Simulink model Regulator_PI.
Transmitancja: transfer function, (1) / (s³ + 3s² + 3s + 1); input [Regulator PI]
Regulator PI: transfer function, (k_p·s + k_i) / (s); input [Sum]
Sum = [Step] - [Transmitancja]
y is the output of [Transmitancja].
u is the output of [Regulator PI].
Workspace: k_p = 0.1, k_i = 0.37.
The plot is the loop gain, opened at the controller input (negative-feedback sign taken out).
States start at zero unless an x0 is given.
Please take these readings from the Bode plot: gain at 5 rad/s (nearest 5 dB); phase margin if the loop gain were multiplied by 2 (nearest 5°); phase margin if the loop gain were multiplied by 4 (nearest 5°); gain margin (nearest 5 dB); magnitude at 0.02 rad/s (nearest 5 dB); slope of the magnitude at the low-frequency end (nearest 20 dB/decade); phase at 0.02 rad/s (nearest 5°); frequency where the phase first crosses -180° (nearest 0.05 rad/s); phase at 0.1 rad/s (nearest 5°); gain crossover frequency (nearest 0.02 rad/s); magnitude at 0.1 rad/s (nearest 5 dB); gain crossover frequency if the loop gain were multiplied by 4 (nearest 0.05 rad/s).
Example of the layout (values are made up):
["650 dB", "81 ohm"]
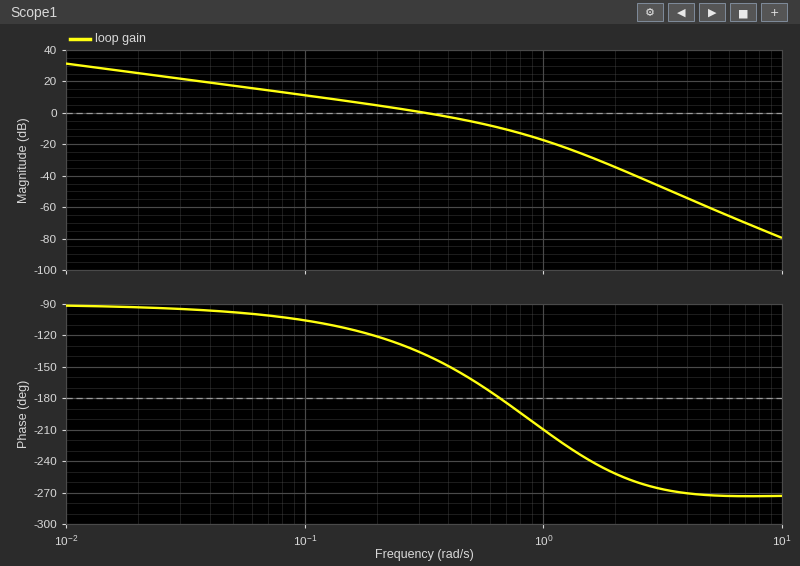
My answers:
["-60 dB", "15°", "-10°", "10 dB", "25 dB", "-20 dB/decade", "-95°", "0.65 rad/s", "-105°", "0.32 rad/s", "10 dB", "0.75 rad/s"]
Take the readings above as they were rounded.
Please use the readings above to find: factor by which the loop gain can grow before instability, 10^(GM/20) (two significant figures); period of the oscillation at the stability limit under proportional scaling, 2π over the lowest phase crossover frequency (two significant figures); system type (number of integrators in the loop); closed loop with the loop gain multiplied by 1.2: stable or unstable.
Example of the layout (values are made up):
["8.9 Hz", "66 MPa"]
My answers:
["3.2", "9.7 s", "1", "stable"]
